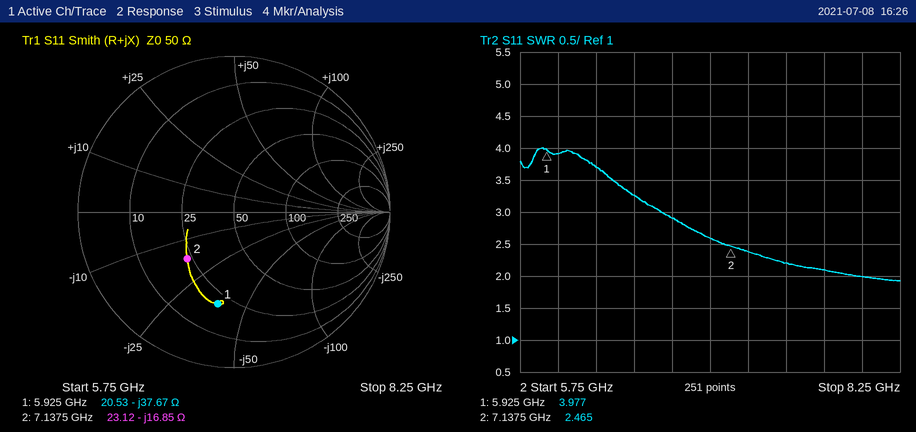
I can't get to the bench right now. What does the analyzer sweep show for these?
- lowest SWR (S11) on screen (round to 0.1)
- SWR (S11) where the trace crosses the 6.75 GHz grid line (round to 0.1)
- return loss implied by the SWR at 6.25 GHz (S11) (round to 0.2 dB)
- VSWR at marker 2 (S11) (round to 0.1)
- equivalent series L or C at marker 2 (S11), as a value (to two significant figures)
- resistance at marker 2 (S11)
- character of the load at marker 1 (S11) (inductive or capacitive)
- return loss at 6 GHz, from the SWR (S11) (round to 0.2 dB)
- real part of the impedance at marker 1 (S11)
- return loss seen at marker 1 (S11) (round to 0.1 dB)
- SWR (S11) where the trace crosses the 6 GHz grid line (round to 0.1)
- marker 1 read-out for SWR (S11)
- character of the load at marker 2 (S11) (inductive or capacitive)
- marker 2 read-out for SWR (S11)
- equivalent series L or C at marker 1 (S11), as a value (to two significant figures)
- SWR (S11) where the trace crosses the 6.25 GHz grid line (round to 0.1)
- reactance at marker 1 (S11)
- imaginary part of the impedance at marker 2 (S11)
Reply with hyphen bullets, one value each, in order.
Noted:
- 1.9
- 2.9
- 4.8 dB
- 2.5
- 1.3 pF
- 23.12 Ω
- capacitive
- 4.6 dB
- 20.53 Ω
- 4.5 dB
- 3.9
- 3.977
- capacitive
- 2.465
- 710 fF
- 3.7
- -37.67 Ω
- -16.85 Ω
